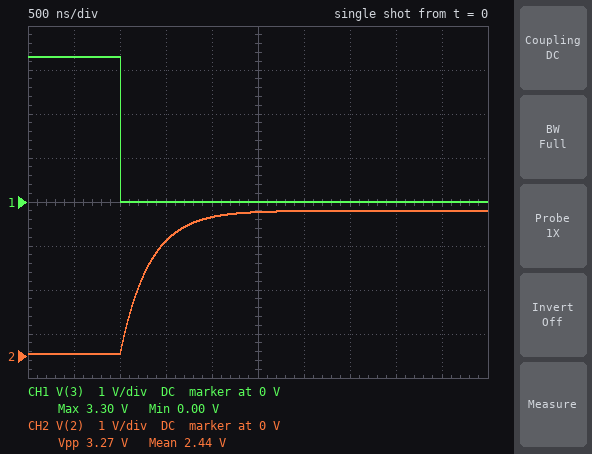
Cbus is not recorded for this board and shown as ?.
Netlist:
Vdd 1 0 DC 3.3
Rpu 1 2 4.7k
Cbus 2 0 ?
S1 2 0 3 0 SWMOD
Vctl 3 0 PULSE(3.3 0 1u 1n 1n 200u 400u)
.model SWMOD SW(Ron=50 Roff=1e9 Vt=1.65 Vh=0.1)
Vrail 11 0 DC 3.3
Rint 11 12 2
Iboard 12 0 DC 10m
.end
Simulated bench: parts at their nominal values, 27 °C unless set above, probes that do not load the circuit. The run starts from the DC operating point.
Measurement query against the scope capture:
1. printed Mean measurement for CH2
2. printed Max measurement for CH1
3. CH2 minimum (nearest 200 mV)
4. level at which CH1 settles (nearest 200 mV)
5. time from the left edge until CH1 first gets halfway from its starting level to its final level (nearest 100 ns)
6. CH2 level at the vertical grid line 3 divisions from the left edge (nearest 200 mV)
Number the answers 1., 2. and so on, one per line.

1. 2.44 V
2. 3.30 V
3. 0 V
4. 0 V
5. 1.0 µs
6. 2.6 V
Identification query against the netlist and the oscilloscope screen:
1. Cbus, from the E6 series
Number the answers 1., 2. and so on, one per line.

1. 68 pF
